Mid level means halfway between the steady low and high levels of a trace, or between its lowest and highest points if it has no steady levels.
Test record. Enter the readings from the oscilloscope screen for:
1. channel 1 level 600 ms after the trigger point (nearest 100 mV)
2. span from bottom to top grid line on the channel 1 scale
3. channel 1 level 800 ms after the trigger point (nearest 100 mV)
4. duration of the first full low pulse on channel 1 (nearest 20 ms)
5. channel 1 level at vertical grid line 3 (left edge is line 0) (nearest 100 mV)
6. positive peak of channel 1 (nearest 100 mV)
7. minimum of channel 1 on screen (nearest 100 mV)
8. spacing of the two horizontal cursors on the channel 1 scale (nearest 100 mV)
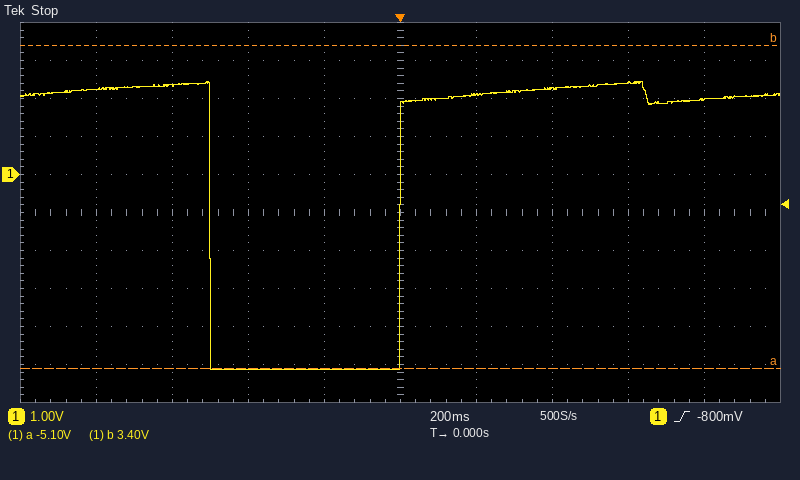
2.4 V
10 V
2.0 V
500 ms
-5.1 V
2.4 V
-5.1 V
8.5 V
